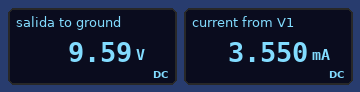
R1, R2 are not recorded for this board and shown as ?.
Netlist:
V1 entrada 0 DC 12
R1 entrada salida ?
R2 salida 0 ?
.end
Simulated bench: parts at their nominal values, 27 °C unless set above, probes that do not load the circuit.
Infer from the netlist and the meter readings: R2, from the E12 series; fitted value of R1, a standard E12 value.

2.7 kΩ
680 Ω
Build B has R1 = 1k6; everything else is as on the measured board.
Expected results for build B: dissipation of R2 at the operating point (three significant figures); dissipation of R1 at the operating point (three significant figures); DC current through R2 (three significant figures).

21.0 mW
12.5 mW
2.79 mA
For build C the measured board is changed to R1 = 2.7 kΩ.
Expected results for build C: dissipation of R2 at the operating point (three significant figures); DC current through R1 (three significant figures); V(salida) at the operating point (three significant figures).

13.3 mW
2.22 mA
6.00 V
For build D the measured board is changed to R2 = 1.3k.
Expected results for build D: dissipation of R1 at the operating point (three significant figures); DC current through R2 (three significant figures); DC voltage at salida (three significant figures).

25.0 mW
6.06 mA
7.88 V
